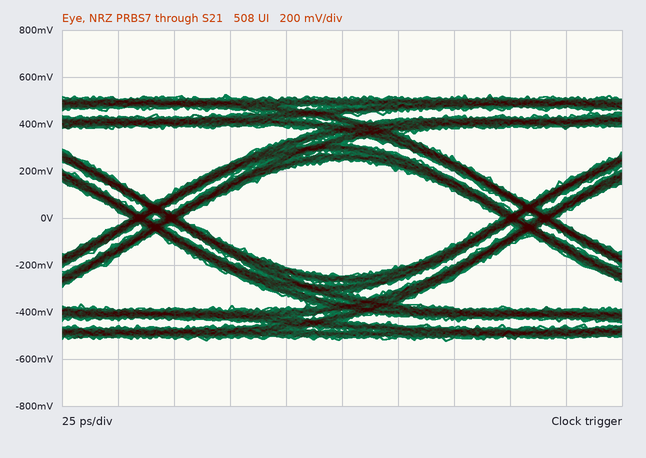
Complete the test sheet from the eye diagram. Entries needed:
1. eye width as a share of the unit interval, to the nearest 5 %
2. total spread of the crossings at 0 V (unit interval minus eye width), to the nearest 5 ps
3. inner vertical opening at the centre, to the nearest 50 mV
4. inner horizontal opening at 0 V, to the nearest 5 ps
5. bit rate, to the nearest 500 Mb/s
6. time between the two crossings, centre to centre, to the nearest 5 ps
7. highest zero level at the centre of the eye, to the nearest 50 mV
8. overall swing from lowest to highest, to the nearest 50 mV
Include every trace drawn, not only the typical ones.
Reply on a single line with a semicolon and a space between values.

85 %; 25 ps; 500 mV; 140 ps; 6.0 Gb/s; 165 ps; -250 mV; 1.05 V
